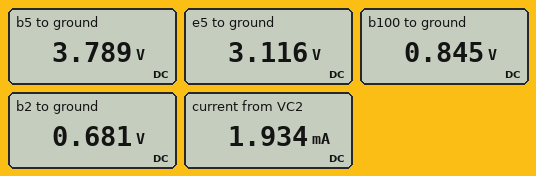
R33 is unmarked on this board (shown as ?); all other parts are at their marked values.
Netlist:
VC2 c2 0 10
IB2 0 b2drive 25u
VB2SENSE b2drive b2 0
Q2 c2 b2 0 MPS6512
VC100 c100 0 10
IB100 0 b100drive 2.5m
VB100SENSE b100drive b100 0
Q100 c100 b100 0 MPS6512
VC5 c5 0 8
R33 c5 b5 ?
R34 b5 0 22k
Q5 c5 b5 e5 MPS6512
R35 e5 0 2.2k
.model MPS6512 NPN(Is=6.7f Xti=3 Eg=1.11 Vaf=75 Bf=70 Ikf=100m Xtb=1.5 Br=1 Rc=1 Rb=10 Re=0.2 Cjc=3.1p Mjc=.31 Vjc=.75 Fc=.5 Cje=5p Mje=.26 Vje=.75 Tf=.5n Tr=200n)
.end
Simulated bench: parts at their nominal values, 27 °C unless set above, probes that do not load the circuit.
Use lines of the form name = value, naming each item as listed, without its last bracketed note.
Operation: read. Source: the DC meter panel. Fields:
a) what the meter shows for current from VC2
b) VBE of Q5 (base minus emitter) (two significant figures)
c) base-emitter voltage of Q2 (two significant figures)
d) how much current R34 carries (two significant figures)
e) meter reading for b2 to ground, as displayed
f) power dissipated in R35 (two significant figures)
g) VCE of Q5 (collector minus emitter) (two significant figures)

what the meter shows for current from VC2 = 1.934 mA
VBE of Q5 (base minus emitter) = 670 mV
base-emitter voltage of Q2 = 680 mV
how much current R34 carries = 170 µA
meter reading for b2 to ground, as displayed = 0.681 V
power dissipated in R35 = 4.4 mW
VCE of Q5 (collector minus emitter) = 4.9 V
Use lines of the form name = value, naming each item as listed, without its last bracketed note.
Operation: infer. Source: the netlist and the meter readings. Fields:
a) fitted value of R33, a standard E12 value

fitted value of R33, a standard E12 value = 22 kΩ
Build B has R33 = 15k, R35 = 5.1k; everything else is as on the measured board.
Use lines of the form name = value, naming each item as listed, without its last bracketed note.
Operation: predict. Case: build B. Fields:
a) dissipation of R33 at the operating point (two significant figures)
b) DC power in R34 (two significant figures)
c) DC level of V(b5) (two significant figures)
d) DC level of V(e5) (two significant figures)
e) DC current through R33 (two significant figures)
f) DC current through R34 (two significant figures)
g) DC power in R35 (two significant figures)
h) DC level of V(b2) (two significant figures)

dissipation of R33 at the operating point = 740 µW
DC power in R34 = 990 µW
DC level of V(b5) = 4.7 V
DC level of V(e5) = 4.0 V
DC current through R33 = 220 µA
DC current through R34 = 210 µA
DC power in R35 = 3.1 mW
DC level of V(b2) = 680 mV
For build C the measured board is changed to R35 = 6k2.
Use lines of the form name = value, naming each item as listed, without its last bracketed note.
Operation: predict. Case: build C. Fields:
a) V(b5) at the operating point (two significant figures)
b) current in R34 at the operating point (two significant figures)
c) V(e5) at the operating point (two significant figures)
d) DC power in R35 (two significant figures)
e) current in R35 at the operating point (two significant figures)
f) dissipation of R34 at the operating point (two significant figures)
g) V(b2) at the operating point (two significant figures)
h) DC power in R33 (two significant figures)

V(b5) at the operating point = 3.9 V
current in R34 at the operating point = 180 µA
V(e5) at the operating point = 3.3 V
DC power in R35 = 1.7 mW
current in R35 at the operating point = 530 µA
dissipation of R34 at the operating point = 700 µW
V(b2) at the operating point = 680 mV
DC power in R33 = 760 µW
